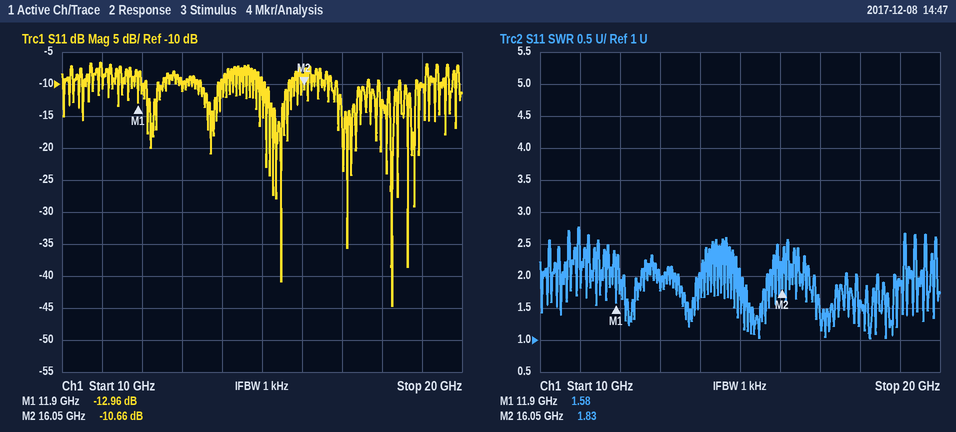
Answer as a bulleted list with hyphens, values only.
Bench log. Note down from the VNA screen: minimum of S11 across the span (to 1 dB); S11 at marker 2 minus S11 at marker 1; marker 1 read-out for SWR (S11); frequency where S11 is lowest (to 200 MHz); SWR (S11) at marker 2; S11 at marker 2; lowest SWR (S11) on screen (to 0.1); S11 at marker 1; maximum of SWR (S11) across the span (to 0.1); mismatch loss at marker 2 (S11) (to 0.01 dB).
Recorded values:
- -45 dB
- 2.30 dB
- 1.58
- 18.2 GHz
- 1.83
- -10.66 dB
- 1.0
- -12.96 dB
- 2.8
- 0.39 dB
